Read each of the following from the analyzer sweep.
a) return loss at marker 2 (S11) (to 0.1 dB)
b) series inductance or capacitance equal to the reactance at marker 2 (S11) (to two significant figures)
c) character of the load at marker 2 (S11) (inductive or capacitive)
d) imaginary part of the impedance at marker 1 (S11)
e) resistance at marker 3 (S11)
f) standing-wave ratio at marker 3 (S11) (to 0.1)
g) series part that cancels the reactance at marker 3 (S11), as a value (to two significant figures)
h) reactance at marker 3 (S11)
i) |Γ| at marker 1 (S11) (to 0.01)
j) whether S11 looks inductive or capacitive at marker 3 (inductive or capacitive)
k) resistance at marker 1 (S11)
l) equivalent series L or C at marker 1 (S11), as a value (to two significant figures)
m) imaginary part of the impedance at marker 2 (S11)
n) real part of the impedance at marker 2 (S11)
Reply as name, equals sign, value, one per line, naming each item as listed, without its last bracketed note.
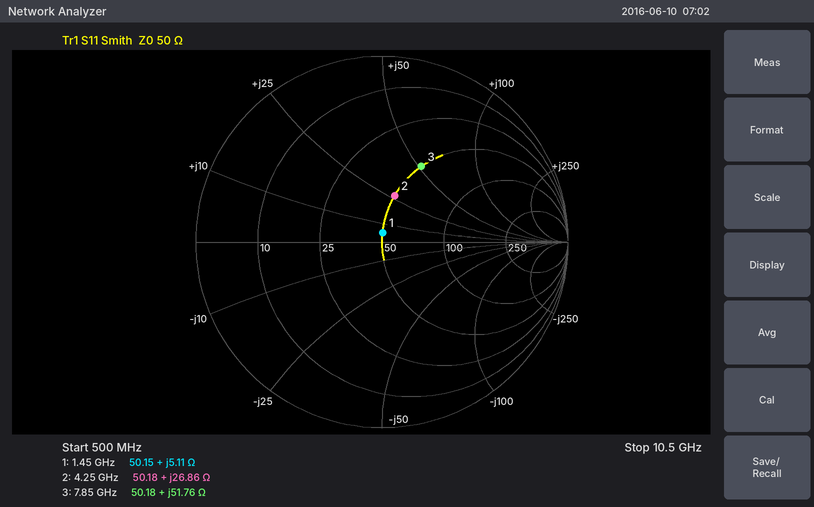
return loss at marker 2 (S11) = 11.7 dB
series inductance or capacitance equal to the reactance at marker 2 (S11) = 1.0 nH
character of the load at marker 2 (S11) = inductive
imaginary part of the impedance at marker 1 = +5.11 Ω
resistance at marker 3 = 50.18 Ω
standing-wave ratio at marker 3 (S11) = 2.7
series part that cancels the reactance at marker 3 (S11), as a value = 390 fF
reactance at marker 3 = +51.76 Ω
|Γ| at marker 1 (S11) = 0.05
whether S11 looks inductive or capacitive at marker 3 = inductive
resistance at marker 1 = 50.15 Ω
equivalent series L or C at marker 1 (S11), as a value = 560 pH
imaginary part of the impedance at marker 2 = +26.86 Ω
real part of the impedance at marker 2 = 50.18 Ω
